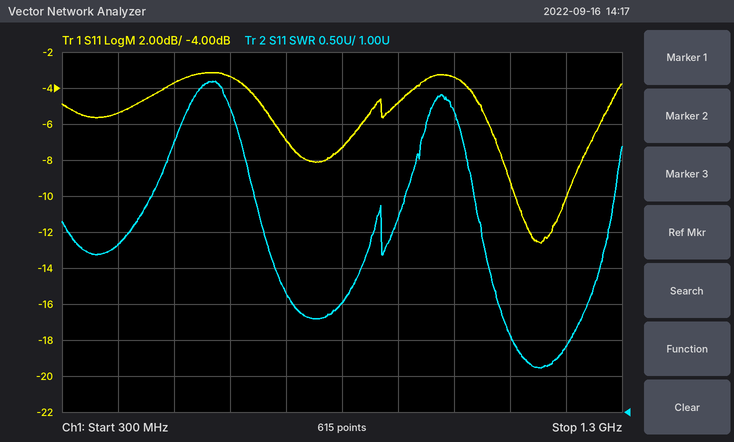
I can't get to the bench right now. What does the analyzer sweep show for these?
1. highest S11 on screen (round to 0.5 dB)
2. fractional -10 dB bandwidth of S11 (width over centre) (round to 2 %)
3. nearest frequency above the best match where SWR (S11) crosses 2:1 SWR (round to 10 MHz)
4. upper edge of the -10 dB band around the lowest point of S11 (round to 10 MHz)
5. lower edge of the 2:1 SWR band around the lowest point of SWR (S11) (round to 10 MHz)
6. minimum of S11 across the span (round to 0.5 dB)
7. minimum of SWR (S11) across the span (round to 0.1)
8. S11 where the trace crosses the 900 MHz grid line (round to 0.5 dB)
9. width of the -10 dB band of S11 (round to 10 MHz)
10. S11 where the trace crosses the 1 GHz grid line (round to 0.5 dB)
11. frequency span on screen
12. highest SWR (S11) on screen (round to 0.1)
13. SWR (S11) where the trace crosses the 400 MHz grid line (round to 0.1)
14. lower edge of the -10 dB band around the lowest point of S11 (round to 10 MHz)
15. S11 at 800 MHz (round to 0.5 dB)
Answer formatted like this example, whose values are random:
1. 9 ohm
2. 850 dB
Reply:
1. -3.0 dB
2. 8 %
3. 1.21 GHz
4. 1.20 GHz
5. 1.10 GHz
6. -12.5 dB
7. 1.6
8. -5.0 dB
9. 90 MHz
10. -3.5 dB
11. 1 GHz
12. 5.6
13. 3.3
14. 1.11 GHz
15. -7.5 dB
